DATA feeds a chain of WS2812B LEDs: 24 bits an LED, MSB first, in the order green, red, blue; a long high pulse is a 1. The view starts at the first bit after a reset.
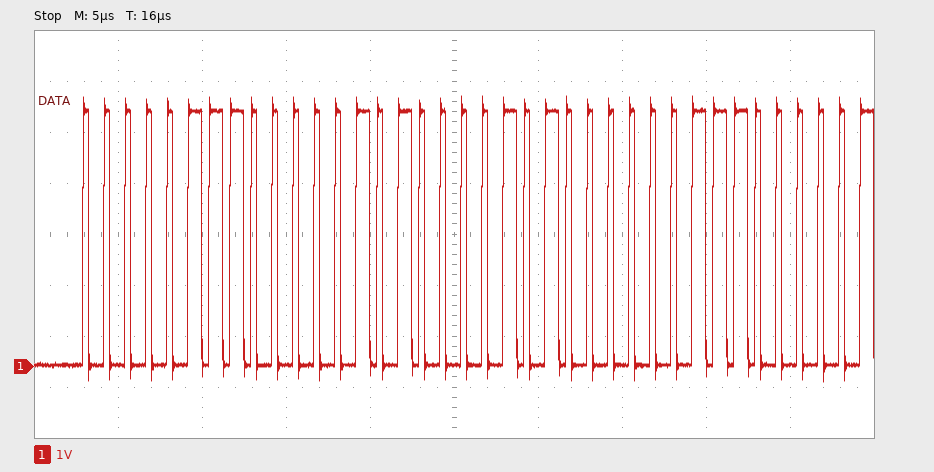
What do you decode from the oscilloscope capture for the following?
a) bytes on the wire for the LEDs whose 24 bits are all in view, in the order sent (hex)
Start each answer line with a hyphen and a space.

- 07 05 0A
